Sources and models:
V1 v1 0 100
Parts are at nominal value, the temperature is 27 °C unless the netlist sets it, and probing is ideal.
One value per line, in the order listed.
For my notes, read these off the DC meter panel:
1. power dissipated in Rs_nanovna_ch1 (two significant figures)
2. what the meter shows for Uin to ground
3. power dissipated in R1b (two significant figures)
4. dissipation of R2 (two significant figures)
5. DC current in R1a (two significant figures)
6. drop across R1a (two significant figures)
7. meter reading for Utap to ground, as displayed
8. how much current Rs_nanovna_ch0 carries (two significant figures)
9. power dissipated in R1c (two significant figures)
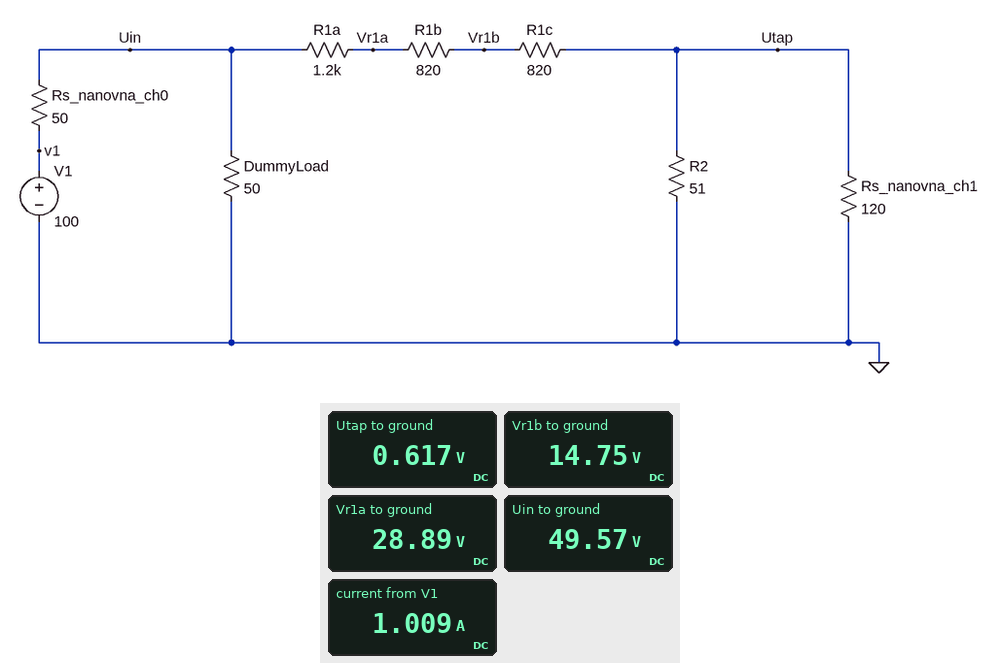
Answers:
3.2 mW
49.57 V
240 mW
7.5 mW
17 mA
21 V
0.617 V
1.0 A
240 mW
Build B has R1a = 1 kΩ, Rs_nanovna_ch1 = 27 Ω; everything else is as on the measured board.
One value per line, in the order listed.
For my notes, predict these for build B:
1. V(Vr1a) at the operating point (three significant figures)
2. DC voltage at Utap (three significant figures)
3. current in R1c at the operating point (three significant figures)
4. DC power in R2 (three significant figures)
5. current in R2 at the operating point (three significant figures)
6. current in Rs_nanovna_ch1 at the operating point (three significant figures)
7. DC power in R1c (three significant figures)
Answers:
30.9 V
329 mV
18.6 mA
2.12 mW
6.45 mA
12.2 mA
285 mW
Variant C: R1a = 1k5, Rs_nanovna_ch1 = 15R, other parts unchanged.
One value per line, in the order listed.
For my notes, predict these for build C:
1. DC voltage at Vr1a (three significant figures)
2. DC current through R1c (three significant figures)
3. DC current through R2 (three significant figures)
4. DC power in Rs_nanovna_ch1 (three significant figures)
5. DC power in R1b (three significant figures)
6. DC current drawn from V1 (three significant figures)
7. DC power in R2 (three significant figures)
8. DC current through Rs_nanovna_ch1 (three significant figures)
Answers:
26.0 V
15.7 mA
3.58 mA
2.22 mW
203 mW
1.01 A
653 µW
12.2 mA
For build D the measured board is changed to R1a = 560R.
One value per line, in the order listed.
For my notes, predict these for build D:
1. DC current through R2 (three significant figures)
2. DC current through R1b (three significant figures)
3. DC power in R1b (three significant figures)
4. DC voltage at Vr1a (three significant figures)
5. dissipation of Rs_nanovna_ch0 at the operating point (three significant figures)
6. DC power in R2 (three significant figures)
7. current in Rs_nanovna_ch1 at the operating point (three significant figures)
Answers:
15.5 mA
22.1 mA
401 mW
37.1 V
51.1 W
12.3 mW
6.60 mA
